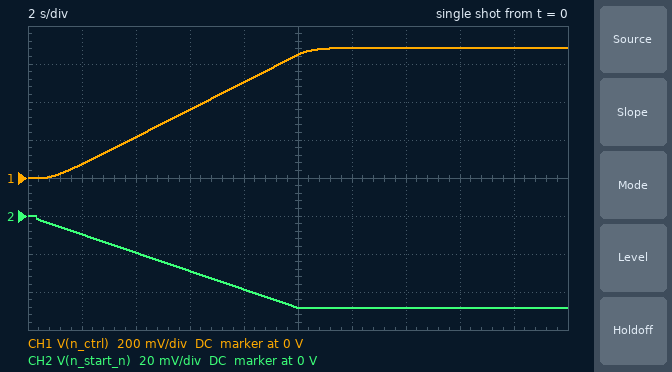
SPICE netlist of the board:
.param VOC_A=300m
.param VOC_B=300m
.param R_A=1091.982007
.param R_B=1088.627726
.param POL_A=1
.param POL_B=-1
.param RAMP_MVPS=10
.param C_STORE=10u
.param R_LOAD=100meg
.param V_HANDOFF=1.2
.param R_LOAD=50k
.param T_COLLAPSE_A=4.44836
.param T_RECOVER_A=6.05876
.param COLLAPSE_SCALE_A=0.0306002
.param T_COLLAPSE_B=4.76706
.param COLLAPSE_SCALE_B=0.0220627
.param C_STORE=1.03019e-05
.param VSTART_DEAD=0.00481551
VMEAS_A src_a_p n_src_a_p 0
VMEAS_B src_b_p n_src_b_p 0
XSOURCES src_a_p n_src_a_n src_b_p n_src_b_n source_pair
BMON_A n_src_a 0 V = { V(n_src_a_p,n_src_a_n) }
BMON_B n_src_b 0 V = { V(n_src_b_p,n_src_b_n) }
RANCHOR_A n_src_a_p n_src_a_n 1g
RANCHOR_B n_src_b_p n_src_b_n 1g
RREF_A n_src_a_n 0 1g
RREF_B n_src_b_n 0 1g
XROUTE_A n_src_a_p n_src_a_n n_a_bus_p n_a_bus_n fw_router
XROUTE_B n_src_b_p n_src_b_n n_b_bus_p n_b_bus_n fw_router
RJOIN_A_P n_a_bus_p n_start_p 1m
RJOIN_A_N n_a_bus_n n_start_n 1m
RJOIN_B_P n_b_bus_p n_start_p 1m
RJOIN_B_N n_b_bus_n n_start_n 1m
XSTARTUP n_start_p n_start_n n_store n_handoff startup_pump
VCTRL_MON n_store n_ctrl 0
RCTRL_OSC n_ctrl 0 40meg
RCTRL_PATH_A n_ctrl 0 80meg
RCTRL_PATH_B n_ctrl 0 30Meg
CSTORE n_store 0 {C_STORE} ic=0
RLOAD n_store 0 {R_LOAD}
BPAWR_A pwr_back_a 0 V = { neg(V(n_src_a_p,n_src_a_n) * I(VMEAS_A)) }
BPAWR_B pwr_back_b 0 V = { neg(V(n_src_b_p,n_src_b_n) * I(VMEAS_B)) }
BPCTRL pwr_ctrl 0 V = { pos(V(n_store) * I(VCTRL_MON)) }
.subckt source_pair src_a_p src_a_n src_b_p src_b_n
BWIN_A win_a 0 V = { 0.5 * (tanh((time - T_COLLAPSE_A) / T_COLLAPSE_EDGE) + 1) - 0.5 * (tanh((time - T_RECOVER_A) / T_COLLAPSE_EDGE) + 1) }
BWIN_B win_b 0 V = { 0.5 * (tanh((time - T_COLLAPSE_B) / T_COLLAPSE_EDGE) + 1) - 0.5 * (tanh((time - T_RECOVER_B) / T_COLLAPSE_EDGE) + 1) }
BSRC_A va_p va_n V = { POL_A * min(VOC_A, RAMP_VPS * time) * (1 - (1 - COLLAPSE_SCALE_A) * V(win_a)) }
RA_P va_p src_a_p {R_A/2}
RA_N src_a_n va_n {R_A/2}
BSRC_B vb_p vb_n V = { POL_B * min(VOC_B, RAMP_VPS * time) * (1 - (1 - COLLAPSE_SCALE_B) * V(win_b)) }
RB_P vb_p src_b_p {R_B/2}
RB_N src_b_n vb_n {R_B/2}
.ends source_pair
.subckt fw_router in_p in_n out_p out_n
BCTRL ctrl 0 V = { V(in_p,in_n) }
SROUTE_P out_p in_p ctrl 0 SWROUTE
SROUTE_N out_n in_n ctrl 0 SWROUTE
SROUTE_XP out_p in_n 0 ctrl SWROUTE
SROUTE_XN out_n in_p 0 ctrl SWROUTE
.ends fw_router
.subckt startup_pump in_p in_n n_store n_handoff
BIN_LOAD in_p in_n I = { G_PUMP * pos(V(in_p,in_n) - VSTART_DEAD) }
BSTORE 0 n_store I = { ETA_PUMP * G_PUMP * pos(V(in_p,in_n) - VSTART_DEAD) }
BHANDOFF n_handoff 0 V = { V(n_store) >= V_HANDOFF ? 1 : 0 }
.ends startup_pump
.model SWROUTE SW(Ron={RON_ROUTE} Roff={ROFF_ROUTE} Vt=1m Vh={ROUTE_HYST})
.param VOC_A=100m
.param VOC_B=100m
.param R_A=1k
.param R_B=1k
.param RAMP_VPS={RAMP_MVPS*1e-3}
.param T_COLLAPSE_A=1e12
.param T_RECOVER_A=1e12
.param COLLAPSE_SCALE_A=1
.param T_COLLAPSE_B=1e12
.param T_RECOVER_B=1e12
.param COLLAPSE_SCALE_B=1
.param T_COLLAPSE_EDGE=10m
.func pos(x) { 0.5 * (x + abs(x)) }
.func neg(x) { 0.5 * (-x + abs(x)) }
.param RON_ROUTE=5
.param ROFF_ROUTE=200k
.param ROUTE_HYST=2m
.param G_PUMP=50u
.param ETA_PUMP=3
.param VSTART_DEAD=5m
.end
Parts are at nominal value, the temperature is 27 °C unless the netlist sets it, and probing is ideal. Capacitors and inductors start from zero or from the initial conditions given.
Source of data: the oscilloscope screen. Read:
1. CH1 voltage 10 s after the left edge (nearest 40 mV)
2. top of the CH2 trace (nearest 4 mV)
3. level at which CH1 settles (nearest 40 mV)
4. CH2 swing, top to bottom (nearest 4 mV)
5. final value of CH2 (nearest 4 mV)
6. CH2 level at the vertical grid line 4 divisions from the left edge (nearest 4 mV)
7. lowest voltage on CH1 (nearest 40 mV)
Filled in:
640 mV
0 V
680 mV
48 mV
-48 mV
-40 mV
0 V
